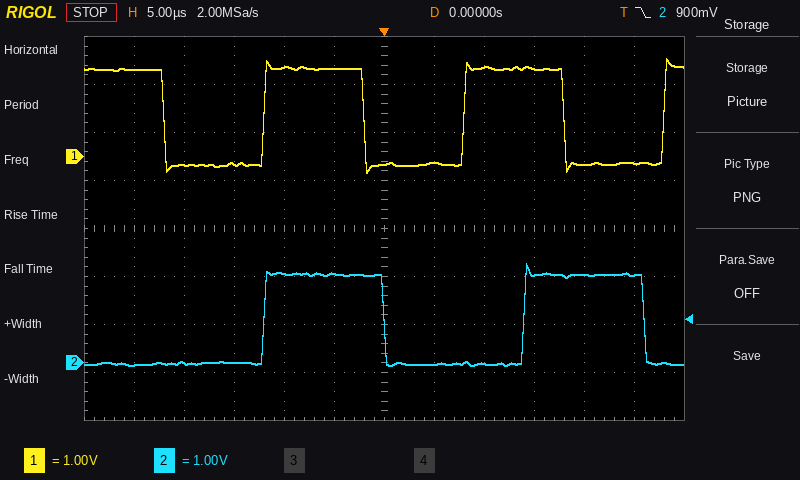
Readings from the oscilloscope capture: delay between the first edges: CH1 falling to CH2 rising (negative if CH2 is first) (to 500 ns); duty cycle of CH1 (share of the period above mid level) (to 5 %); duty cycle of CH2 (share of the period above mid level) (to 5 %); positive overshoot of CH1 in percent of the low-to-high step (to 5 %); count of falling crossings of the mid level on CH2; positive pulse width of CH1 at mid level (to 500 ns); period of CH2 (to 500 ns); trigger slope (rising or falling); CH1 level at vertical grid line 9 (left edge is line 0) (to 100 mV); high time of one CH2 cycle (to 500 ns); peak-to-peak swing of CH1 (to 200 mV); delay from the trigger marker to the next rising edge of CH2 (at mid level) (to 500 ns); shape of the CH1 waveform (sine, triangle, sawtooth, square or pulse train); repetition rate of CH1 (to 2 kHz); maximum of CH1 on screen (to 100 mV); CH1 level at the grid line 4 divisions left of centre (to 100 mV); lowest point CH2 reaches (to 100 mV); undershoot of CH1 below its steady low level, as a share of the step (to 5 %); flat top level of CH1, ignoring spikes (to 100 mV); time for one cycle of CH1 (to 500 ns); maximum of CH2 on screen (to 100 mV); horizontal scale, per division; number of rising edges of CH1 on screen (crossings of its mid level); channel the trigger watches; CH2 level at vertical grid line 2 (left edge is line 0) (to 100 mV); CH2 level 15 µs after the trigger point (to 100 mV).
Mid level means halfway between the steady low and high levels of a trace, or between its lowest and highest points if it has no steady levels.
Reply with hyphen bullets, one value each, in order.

- +10.0 µs
- 50 %
- 45 %
- 10 %
- 2
- 10.0 µs
- 26.0 µs
- falling
- 1.8 V
- 12.0 µs
- 2.4 V
- 14.0 µs
- square
- 50 kHz
- 2.0 V
- -200 mV
- -100 mV
- 10 %
- 1.8 V
- 20.0 µs
- 2.1 V
- 5 µs
- 3
- CH2
- 0.0 V
- 1.8 V
